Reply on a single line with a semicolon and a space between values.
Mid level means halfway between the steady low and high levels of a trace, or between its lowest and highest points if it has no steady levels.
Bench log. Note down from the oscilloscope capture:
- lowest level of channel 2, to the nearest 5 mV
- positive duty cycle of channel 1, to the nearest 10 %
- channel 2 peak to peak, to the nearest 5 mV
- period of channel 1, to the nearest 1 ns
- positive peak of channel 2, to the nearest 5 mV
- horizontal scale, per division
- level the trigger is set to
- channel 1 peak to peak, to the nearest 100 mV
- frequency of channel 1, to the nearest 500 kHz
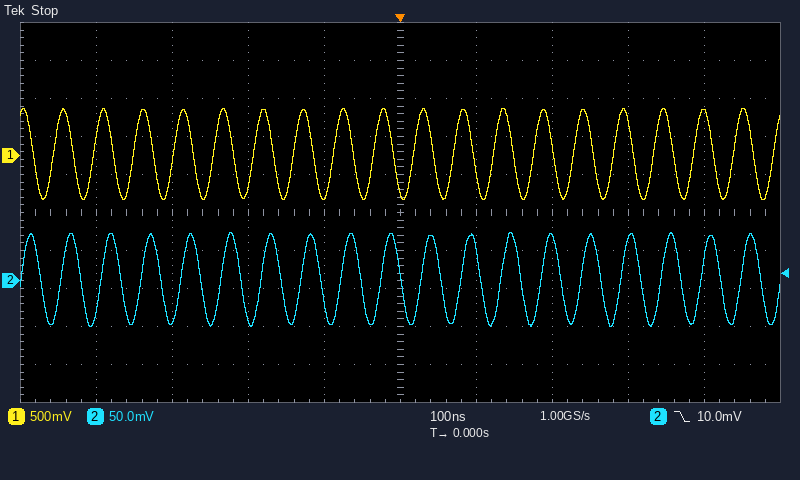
-60 mV; 50 %; 125 mV; 53 ns; 65 mV; 100 ns; 10.0 mV; 1.20 V; 19.0 MHz
